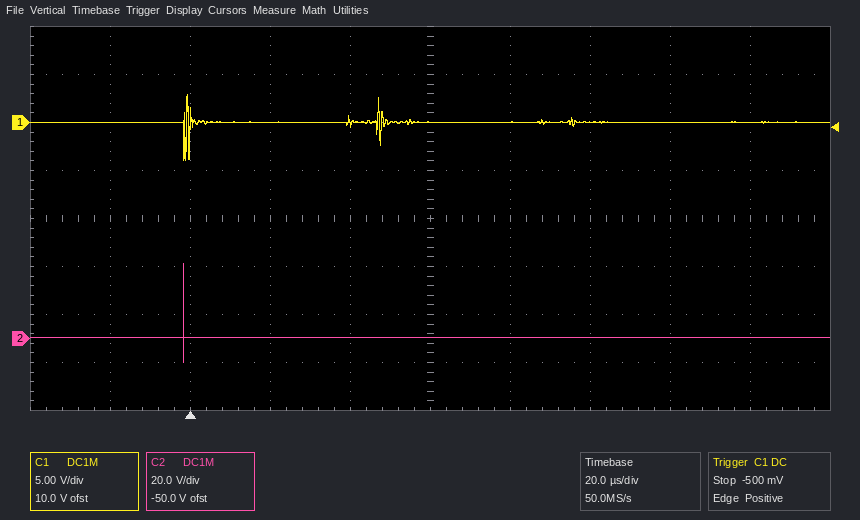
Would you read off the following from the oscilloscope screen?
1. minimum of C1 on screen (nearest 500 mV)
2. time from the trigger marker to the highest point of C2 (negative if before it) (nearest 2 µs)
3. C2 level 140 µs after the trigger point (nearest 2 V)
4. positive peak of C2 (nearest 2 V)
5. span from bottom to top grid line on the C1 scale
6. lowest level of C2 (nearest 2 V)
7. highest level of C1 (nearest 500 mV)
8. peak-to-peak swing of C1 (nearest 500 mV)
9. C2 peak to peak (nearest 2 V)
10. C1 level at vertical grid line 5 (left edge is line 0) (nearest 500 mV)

-4.0 V
-2 µs
0 V
32 V
40 V
-10 V
3.0 V
7.0 V
42 V
0.0 V
